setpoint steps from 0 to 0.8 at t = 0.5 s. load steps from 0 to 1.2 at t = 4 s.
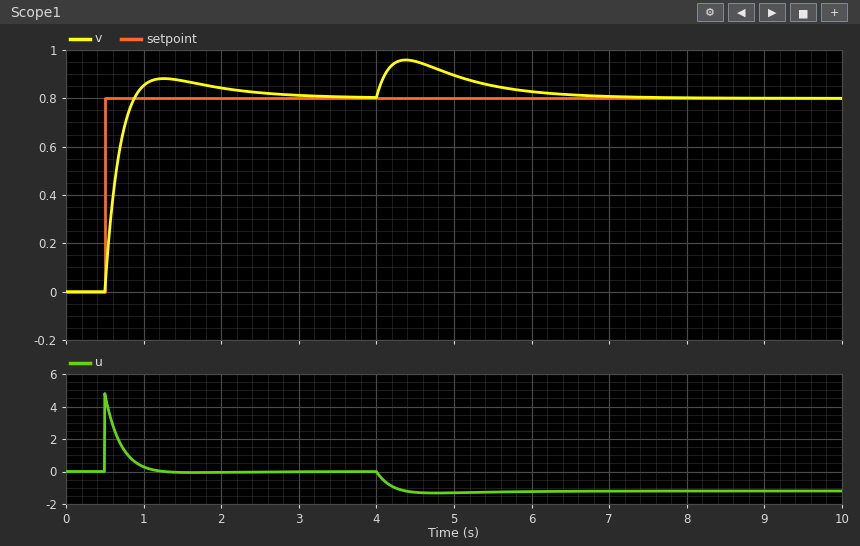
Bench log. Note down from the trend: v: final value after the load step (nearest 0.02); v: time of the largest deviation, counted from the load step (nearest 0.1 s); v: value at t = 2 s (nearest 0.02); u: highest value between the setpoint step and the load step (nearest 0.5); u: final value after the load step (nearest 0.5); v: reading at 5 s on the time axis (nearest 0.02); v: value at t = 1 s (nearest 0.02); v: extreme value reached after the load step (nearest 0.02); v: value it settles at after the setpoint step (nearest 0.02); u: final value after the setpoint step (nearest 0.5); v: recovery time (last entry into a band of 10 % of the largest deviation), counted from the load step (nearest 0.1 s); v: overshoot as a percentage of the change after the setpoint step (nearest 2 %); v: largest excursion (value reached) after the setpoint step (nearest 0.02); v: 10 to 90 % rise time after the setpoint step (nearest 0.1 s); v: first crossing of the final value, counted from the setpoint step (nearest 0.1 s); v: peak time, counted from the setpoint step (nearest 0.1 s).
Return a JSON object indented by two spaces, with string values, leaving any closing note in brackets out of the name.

{
  "v: final value after the load step": "0.80",
  "v: time of the largest deviation, counted from the load step": "0.4 s",
  "v: value at t = 2 s": "0.84",
  "u: highest value between the setpoint step and the load step": "5.0",
  "u: final value after the load step": "-1.0",
  "v: reading at 5 s on the time axis": "0.90",
  "v: value at t = 1 s": "0.86",
  "v: extreme value reached after the load step": "0.96",
  "v: value it settles at after the setpoint step": "0.80",
  "u: final value after the setpoint step": "0.0",
  "v: recovery time (last entry into a band of 10 % of the largest deviation), counted from the load step": "2.5 s",
  "v: overshoot as a percentage of the change after the setpoint step": "10 %",
  "v: largest excursion (value reached) after the setpoint step": "0.88",
  "v: 10 to 90 % rise time after the setpoint step": "0.3 s",
  "v: first crossing of the final value, counted from the setpoint step": "0.4 s",
  "v: peak time, counted from the setpoint step": "0.8 s"
}
